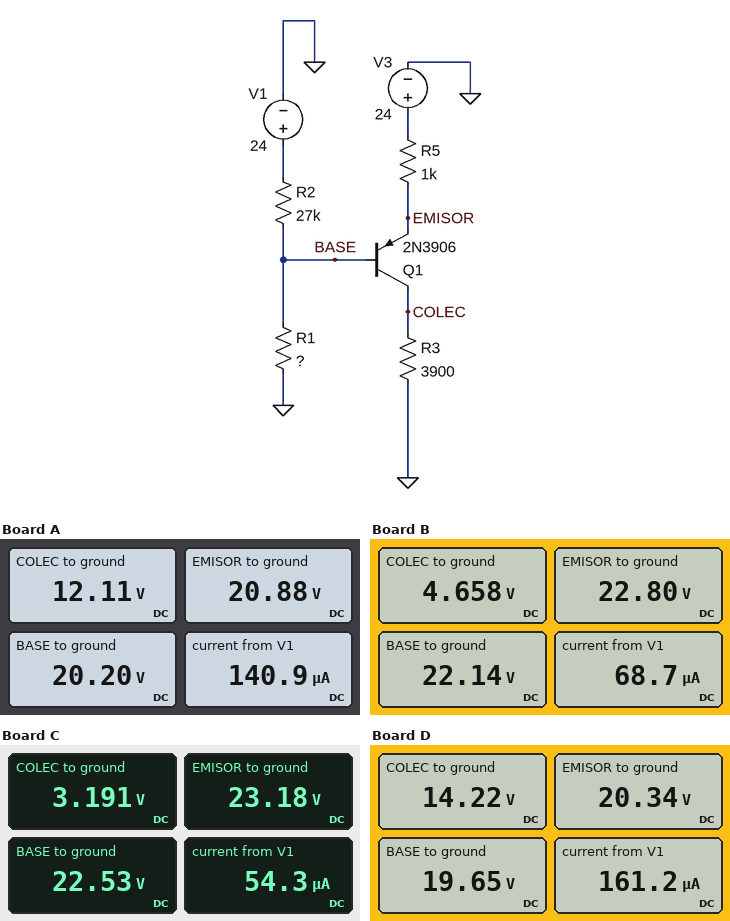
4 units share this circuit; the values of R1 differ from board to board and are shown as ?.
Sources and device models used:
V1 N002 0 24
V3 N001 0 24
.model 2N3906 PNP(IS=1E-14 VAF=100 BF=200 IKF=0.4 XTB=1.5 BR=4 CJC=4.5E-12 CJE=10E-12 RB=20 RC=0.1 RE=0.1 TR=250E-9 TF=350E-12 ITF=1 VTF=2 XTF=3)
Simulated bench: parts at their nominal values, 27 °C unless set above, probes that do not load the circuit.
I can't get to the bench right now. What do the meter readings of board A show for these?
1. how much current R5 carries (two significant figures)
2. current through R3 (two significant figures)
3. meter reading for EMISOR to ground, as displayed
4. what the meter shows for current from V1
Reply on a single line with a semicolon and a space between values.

3.1 mA; 3.1 mA; 20.88 V; 140.9 µA
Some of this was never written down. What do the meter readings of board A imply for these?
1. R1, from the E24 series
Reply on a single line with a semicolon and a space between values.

130 kΩ
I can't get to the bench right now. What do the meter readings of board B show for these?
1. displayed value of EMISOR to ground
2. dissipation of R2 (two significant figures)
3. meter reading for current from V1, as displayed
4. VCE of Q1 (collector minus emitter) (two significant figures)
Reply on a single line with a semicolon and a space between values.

22.80 V; 130 µW; 68.7 µA; -18 V
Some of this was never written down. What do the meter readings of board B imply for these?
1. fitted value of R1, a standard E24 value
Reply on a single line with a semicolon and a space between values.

300 kΩ
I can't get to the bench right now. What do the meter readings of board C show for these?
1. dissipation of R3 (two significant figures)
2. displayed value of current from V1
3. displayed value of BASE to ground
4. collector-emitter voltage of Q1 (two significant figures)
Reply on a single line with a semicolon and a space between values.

2.6 mW; 54.3 µA; 22.53 V; -20 V
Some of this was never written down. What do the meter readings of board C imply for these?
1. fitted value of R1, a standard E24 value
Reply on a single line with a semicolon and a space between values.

390 kΩ
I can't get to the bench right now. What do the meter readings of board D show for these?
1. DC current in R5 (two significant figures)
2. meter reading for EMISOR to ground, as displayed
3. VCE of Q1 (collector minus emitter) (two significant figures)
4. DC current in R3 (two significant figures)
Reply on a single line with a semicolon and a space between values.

3.7 mA; 20.34 V; -6.1 V; 3.6 mA
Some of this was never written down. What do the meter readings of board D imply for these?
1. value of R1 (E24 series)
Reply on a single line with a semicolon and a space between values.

110 kΩ
